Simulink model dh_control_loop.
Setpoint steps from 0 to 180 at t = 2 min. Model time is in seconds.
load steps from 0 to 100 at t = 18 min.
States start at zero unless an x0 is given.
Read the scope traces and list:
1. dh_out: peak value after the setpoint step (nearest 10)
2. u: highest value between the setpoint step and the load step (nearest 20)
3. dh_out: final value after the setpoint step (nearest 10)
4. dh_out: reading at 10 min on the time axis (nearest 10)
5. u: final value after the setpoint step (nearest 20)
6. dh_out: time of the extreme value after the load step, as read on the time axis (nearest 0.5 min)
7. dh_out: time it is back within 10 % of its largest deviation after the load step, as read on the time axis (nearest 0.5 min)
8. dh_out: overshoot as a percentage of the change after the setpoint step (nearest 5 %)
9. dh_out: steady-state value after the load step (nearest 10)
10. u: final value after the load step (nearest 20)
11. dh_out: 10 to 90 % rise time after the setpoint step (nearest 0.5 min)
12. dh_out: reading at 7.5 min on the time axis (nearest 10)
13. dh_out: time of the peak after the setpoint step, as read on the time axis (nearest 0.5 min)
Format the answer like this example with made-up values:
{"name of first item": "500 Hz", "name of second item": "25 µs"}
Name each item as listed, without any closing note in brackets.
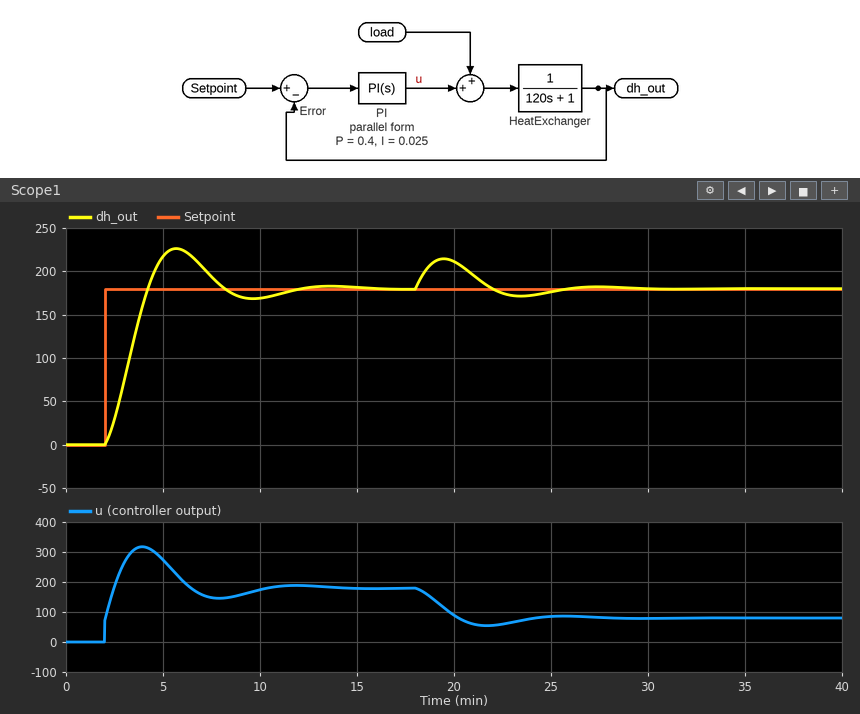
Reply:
{"dh_out: peak value after the setpoint step": "230", "u: highest value between the setpoint step and the load step": "320", "dh_out: final value after the setpoint step": "180", "dh_out: reading at 10 min on the time axis": "170", "u: final value after the setpoint step": "180", "dh_out: time of the extreme value after the load step, as read on the time axis": "19.5 min", "dh_out: time it is back within 10 % of its largest deviation after the load step, as read on the time axis": "25.0 min", "dh_out: overshoot as a percentage of the change after the setpoint step": "25 %", "dh_out: steady-state value after the load step": "180", "u: final value after the load step": "80", "dh_out: 10 to 90 % rise time after the setpoint step": "1.5 min", "dh_out: reading at 7.5 min on the time axis": "190", "dh_out: time of the peak after the setpoint step, as read on the time axis": "5.5 min"}
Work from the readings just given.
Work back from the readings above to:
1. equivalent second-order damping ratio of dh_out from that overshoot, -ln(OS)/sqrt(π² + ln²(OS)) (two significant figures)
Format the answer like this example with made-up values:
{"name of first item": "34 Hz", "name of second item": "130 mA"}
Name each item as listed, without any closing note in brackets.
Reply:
{"equivalent second-order damping ratio of dh_out from that overshoot, -ln(OS)/sqrt(π² + ln²(OS))": "0.40"}
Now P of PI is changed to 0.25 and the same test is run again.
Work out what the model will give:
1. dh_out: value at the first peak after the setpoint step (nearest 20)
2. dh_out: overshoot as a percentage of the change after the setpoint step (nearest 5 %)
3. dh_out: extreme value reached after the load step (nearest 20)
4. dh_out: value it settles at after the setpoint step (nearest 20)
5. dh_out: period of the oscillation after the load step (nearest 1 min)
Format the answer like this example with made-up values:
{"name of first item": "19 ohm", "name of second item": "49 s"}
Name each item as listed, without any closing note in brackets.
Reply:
{"dh_out: value at the first peak after the setpoint step": "240", "dh_out: overshoot as a percentage of the change after the setpoint step": "30 %", "dh_out: extreme value reached after the load step": "220", "dh_out: value it settles at after the setpoint step": "180", "dh_out: period of the oscillation after the load step": "8 min"}
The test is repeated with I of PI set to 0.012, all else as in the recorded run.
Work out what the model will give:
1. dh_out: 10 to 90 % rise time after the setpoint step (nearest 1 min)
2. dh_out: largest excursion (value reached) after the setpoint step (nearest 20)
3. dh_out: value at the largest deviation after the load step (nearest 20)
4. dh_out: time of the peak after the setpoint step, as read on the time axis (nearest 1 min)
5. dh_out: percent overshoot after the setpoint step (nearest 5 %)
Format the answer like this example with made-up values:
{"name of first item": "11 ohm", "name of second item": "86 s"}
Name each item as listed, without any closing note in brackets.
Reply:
{"dh_out: 10 to 90 % rise time after the setpoint step": "3 min", "dh_out: largest excursion (value reached) after the setpoint step": "200", "dh_out: value at the largest deviation after the load step": "220", "dh_out: time of the peak after the setpoint step, as read on the time axis": "8 min", "dh_out: percent overshoot after the setpoint step": "10 %"}
